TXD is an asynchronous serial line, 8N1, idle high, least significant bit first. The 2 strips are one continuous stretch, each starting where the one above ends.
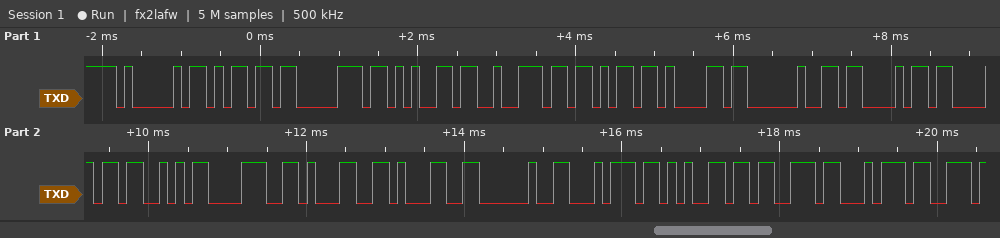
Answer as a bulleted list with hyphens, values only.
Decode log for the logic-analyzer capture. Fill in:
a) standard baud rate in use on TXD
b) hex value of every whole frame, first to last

- 9600 baud
- 41 6D 70 65 72 6B 61 20 43 43 53 38 31 31 20 74 65 73 74
